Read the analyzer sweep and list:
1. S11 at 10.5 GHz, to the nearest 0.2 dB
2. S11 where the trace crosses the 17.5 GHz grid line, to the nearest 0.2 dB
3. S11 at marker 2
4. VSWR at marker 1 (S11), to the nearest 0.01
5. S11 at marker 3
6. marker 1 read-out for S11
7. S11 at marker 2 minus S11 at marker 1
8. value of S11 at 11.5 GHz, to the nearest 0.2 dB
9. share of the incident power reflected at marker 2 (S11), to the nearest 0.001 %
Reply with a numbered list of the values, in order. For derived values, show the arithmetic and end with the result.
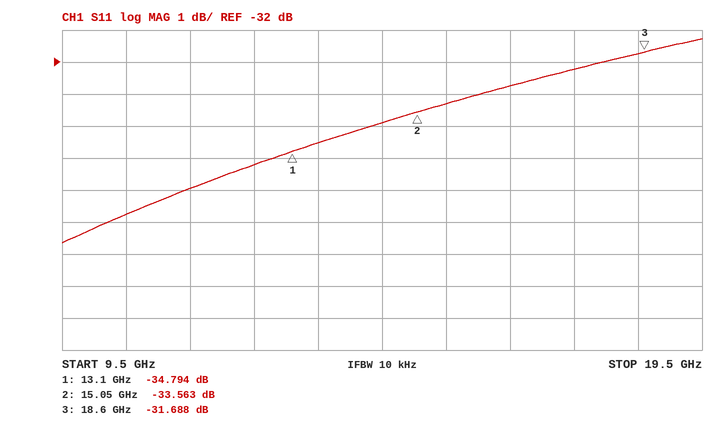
1. -36.8 dB
2. -32.2 dB
3. -33.563 dB
4. (1 + 0.0182)/(1 − 0.0182) ≈ 1.04
5. -31.688 dB
6. -34.794 dB
7. -33.563 − (-34.794) = 1.231 dB
8. -36.0 dB
9. 10^(-33.563/10) ≈ 0.044 %
